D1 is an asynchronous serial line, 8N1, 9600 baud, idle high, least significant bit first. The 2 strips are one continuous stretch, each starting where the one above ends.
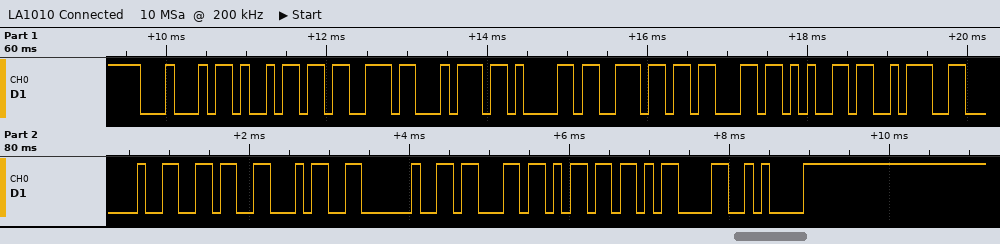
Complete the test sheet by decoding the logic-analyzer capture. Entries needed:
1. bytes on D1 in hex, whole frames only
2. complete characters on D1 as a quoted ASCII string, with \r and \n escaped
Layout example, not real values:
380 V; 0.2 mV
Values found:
44 69 73 74 61 6E 63 65 3A 20 36 34 20 63 6D 0D 0A; "Distance: 64 cm\r\n"
